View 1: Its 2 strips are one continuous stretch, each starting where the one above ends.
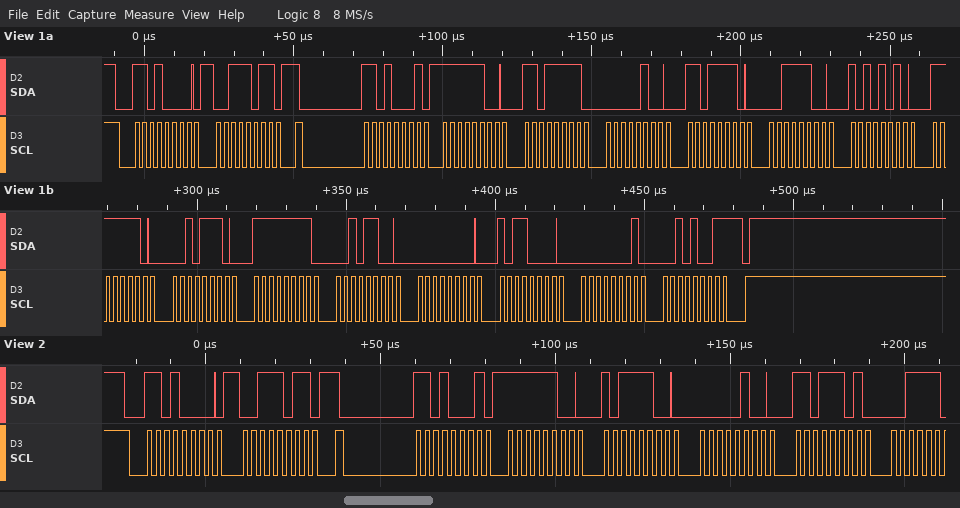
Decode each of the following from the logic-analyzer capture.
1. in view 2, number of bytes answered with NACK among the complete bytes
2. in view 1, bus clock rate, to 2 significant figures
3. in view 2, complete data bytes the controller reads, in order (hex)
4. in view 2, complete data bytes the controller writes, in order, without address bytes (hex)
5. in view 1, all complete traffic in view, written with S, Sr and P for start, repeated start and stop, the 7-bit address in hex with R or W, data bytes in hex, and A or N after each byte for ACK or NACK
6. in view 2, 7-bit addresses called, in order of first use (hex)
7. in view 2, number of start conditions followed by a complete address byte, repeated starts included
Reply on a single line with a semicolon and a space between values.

0; 400 kHz; FC BC 04 DD; 3B; S 68W A 3B A Sr 68R A FC A DF A 04 A DE A 3C A AA A FE A 2E A FF A 2C A 00 A B0 A 01 A 29 N P; 0x68; 2
